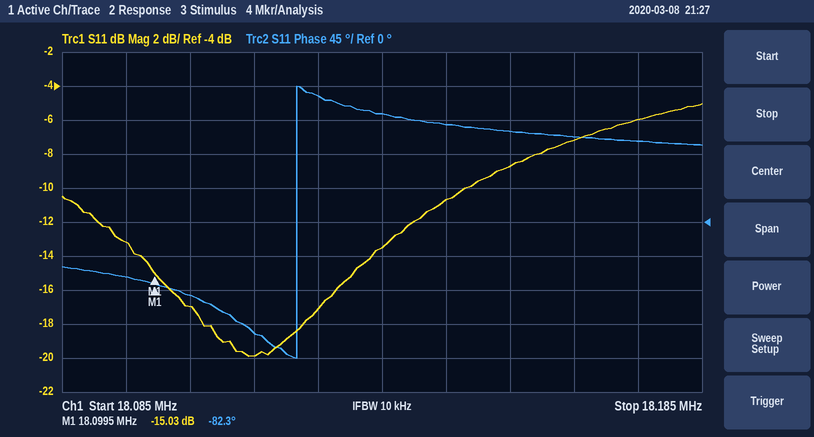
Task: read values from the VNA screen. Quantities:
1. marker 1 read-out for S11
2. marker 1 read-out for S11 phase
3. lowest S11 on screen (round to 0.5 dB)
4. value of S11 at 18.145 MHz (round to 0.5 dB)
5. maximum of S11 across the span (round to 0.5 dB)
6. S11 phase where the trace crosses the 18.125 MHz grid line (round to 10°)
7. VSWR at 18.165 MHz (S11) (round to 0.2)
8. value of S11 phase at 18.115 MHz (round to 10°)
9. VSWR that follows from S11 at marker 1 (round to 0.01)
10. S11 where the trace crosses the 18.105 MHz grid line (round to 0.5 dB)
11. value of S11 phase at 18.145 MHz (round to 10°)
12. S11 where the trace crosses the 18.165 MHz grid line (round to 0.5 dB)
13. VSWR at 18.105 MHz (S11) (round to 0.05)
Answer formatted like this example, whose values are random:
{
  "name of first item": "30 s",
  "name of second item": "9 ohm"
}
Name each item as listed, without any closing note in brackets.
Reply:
{
  "marker 1 read-out for S11": "-15.03 dB",
  "marker 1 read-out for S11 phase": "-82.3°",
  "lowest S11 on screen": "-20.0 dB",
  "value of S11 at 18.145 MHz": "-10.5 dB",
  "maximum of S11 across the span": "-5.0 dB",
  "S11 phase where the trace crosses the 18.125 MHz grid line": "170°",
  "VSWR at 18.165 MHz (S11)": "2.6",
  "value of S11 phase at 18.115 MHz": "-150°",
  "VSWR that follows from S11 at marker 1": "1.43",
  "S11 where the trace crosses the 18.105 MHz grid line": "-17.0 dB",
  "value of S11 phase at 18.145 MHz": "130°",
  "S11 where the trace crosses the 18.165 MHz grid line": "-7.0 dB",
  "VSWR at 18.105 MHz (S11)": "1.35"
}
